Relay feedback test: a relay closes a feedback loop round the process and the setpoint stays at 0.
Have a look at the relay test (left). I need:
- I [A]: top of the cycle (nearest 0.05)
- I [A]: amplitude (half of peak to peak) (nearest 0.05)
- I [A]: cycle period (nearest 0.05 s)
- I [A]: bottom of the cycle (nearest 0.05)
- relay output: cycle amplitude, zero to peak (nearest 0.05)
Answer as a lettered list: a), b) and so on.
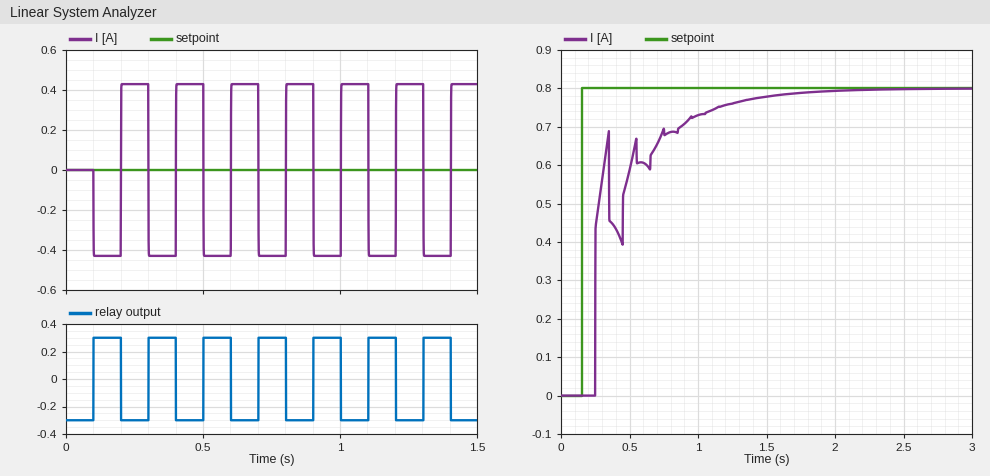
a) 0.45
b) 0.45
c) 0.20 s
d) -0.45
e) 0.30
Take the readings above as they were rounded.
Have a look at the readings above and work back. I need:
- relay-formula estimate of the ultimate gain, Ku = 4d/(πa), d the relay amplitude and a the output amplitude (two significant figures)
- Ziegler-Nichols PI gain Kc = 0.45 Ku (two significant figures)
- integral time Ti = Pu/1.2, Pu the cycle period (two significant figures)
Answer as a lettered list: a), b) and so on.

a) 0.85
b) 0.38
c) 0.17 s
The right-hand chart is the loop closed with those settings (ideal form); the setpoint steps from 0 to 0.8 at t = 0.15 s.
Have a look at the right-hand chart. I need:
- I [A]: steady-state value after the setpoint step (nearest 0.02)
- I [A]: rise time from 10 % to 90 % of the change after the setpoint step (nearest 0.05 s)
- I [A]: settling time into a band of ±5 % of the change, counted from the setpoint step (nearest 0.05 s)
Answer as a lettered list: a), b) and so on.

a) 0.80
b) 0.70 s
c) 1.10 s
